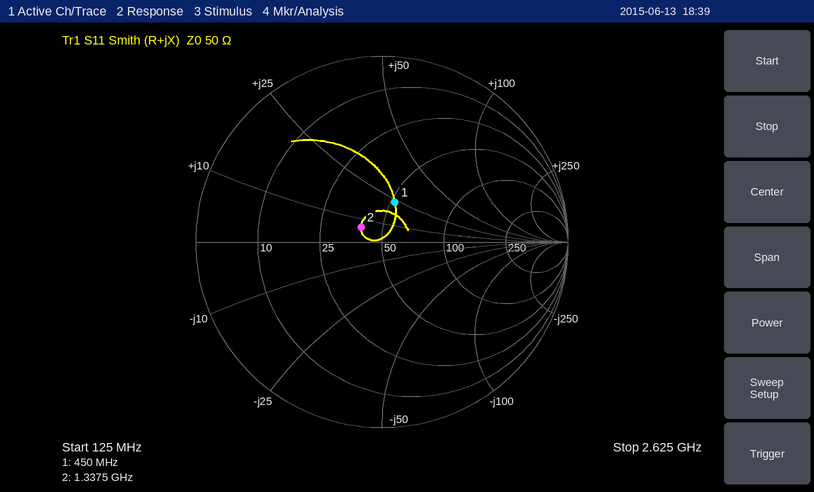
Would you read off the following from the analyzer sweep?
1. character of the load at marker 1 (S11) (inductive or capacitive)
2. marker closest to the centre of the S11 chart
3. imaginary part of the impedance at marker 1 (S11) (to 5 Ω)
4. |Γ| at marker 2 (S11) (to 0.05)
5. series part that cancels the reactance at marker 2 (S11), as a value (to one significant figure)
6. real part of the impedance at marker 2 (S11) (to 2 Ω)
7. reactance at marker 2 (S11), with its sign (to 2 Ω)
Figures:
inductive
marker 2
+25 Ω
0.15
20 pF
40 Ω
+6 Ω
